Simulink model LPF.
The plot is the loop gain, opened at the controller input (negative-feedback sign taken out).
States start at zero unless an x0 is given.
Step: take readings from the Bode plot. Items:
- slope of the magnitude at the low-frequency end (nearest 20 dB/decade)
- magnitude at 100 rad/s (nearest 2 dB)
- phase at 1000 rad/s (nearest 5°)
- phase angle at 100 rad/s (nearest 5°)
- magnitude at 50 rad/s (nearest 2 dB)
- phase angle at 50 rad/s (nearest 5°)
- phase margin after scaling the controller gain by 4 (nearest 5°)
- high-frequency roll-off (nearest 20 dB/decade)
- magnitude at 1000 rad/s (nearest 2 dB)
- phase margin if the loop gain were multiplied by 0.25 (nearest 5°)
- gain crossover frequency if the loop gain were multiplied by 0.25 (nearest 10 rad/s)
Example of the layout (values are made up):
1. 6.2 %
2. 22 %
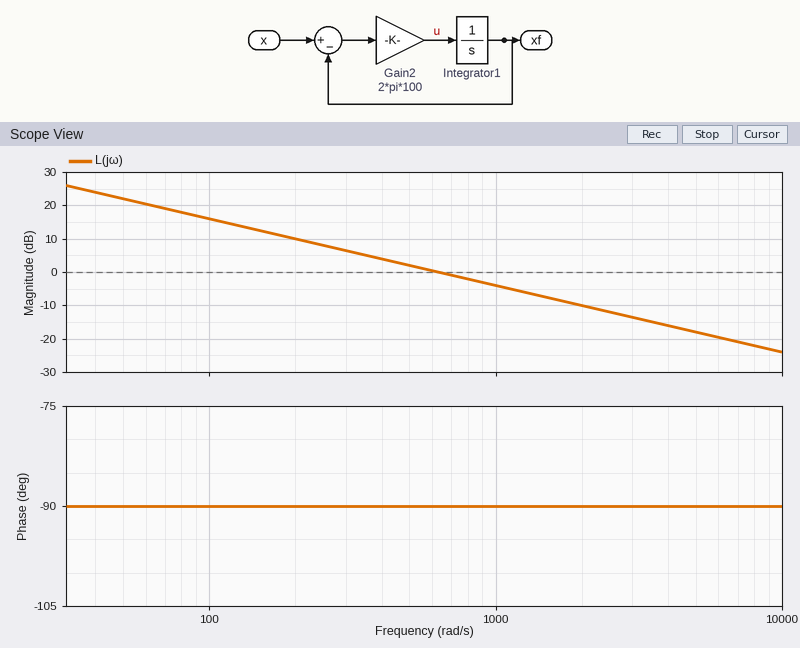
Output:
1. -20 dB/decade
2. 16 dB
3. -90°
4. -90°
5. 22 dB
6. -90°
7. 90°
8. -20 dB/decade
9. -4 dB
10. 90°
11. 160 rad/s
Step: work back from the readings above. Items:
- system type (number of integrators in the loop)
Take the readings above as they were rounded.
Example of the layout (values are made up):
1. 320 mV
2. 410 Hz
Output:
1. 1
